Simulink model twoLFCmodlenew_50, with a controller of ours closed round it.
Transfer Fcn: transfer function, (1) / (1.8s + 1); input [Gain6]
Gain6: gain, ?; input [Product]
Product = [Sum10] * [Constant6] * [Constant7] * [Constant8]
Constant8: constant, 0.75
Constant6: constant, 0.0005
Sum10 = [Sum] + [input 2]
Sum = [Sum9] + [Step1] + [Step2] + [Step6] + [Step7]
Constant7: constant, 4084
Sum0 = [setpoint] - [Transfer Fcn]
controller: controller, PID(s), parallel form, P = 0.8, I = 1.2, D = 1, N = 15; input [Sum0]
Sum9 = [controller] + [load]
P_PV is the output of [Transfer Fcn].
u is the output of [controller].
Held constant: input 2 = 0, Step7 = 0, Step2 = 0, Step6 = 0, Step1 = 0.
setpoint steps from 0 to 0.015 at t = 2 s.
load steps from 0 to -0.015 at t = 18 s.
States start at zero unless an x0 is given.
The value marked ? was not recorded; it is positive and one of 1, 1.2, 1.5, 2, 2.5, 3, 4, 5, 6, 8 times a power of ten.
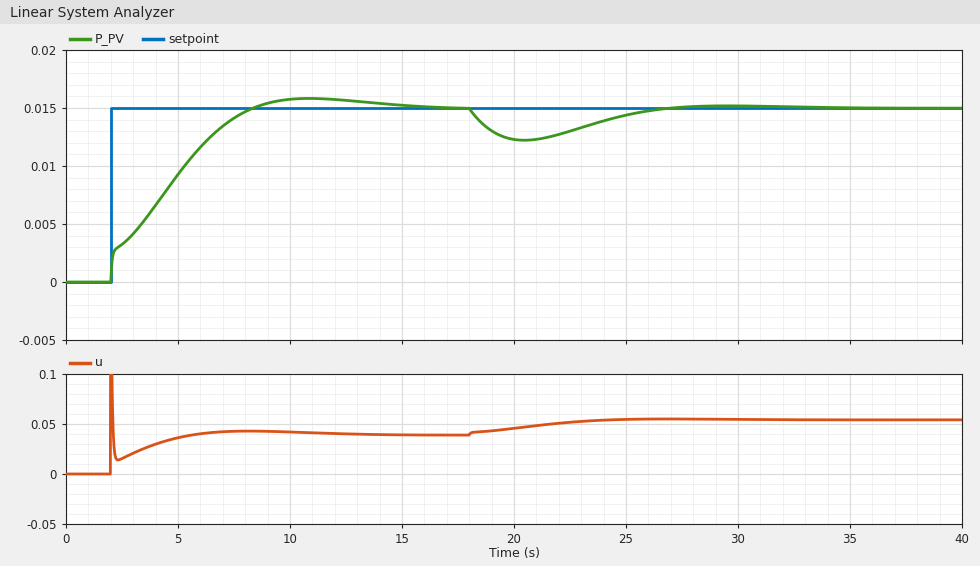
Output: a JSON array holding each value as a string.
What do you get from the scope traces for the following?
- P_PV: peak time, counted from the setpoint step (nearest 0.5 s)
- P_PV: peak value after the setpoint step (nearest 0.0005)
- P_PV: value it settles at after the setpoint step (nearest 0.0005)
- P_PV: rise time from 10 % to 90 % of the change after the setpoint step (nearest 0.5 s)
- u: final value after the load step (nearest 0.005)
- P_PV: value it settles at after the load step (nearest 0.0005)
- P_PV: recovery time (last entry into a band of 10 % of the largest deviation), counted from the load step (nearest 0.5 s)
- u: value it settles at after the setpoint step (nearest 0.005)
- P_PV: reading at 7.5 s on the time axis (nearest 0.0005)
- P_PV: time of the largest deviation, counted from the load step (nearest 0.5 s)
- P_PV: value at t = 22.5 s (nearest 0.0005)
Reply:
["9.0 s", "0.0160", "0.0150", "5.0 s", "0.055", "0.0150", "8.0 s", "0.040", "0.0140", "2.5 s", "0.0130"]
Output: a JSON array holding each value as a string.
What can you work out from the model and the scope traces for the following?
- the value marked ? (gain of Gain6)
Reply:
["0.25"]
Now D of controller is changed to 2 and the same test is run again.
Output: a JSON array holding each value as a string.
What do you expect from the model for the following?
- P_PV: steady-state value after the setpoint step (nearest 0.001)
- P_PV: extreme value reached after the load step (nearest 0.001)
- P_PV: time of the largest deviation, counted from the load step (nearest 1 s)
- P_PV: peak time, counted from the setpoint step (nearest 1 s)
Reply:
["0.015", "0.012", "3 s", "10 s"]
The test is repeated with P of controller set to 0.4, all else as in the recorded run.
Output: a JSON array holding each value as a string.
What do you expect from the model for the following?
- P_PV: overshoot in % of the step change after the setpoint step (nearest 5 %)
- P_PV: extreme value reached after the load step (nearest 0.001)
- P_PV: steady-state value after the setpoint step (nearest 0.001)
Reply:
["10 %", "0.012", "0.015"]
